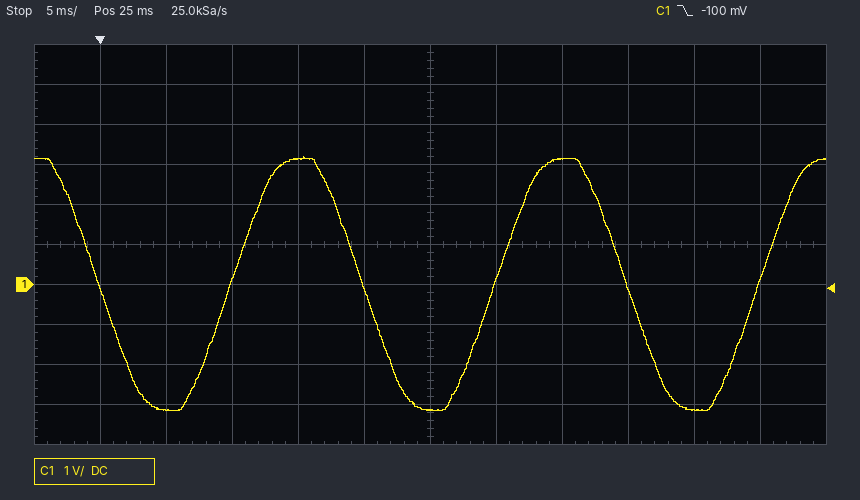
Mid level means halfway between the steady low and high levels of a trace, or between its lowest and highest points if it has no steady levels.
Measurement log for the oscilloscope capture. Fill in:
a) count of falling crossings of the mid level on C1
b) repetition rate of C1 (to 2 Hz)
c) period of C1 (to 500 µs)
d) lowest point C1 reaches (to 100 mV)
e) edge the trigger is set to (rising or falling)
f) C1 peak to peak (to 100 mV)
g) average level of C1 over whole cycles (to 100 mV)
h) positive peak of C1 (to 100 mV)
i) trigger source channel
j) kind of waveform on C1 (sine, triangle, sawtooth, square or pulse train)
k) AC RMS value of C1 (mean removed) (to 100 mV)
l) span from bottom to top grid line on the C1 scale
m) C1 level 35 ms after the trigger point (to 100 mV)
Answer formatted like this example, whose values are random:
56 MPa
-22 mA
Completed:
3
50 Hz
20.0 ms
-3.2 V
falling
6.4 V
0.0 V
3.2 V
C1
sine
2.3 V
10 V
3.1 V
